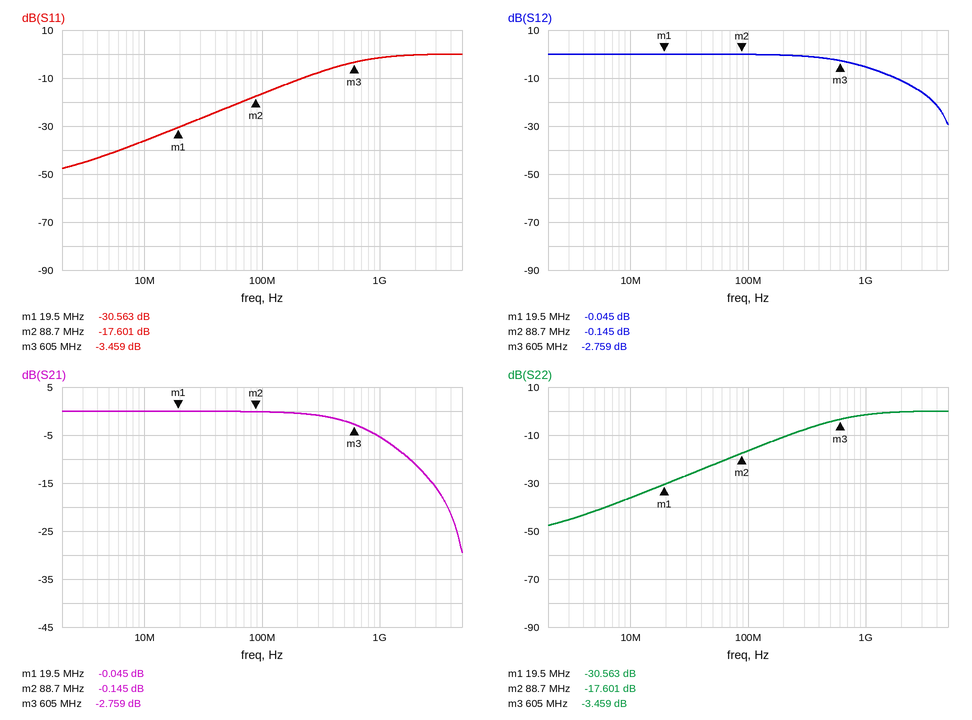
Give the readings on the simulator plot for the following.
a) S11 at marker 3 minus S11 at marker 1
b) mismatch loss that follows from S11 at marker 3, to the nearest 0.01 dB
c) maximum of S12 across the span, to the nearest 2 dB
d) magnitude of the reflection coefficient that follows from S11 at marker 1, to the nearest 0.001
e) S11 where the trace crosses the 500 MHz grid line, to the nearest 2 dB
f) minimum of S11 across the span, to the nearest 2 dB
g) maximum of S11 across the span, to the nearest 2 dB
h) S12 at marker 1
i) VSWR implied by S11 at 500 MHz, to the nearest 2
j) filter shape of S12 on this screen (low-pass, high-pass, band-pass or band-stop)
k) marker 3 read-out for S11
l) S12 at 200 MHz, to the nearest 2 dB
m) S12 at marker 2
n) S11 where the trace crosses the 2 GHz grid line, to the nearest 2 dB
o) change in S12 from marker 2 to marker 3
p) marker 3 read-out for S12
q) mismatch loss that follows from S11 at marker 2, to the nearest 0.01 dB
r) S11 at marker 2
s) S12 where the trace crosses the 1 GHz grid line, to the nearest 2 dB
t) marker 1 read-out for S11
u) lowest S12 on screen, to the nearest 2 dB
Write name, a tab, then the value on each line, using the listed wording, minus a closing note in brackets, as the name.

S11 at marker 3 minus S11 at marker 1	27.104 dB
mismatch loss that follows from S11 at marker 3, to the nearest 0.01 dB	2.60 dB
maximum of S12 across the span, to the nearest 2 dB	0 dB
magnitude of the reflection coefficient that follows from S11 at marker 1, to the nearest 0.001	0.030
S11 where the trace crosses the 500 MHz grid line, to the nearest 2 dB	-4 dB
minimum of S11 across the span, to the nearest 2 dB	-48 dB
maximum of S11 across the span, to the nearest 2 dB	0 dB
S12 at marker 1	-0.045 dB
VSWR implied by S11 at 500 MHz, to the nearest 2	4
filter shape of S12 on this screen	low-pass
marker 3 read-out for S11	-3.459 dB
S12 at 200 MHz, to the nearest 2 dB	0 dB
S12 at marker 2	-0.145 dB
S11 where the trace crosses the 2 GHz grid line, to the nearest 2 dB	0 dB
change in S12 from marker 2 to marker 3	-2.614 dB
marker 3 read-out for S12	-2.759 dB
mismatch loss that follows from S11 at marker 2, to the nearest 0.01 dB	0.08 dB
S11 at marker 2	-17.601 dB
S12 where the trace crosses the 1 GHz grid line, to the nearest 2 dB	-6 dB
marker 1 read-out for S11	-30.563 dB
lowest S12 on screen, to the nearest 2 dB	-30 dB
